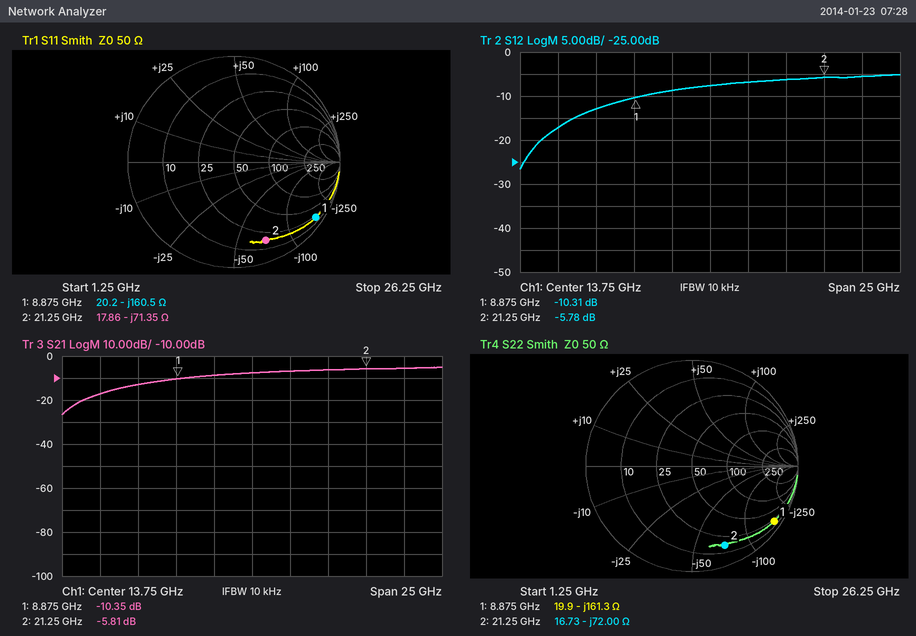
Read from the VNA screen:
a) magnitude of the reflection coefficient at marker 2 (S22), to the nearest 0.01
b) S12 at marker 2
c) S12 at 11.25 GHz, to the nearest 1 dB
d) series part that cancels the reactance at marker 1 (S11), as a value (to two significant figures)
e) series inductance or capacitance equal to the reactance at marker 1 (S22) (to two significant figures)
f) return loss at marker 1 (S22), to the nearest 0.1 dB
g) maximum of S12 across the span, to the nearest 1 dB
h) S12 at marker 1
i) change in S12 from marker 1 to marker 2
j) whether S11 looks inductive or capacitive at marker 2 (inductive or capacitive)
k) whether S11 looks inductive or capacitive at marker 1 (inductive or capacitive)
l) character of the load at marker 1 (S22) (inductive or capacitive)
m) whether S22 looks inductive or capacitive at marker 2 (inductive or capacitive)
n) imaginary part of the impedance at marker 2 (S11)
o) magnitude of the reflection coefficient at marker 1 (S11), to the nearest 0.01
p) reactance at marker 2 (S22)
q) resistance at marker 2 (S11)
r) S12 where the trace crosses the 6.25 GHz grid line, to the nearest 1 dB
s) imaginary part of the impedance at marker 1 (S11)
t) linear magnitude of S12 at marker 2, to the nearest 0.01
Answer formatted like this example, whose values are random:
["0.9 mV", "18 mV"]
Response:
["0.81", "-5.78 dB", "-9 dB", "2.9 nH", "110 fF", "0.6 dB", "-5 dB", "-10.31 dB", "4.53 dB", "capacitive", "capacitive", "capacitive", "capacitive", "-71.35 Ω", "0.93", "-72.00 Ω", "17.86 Ω", "-13 dB", "-160.5 Ω", "0.51"]
